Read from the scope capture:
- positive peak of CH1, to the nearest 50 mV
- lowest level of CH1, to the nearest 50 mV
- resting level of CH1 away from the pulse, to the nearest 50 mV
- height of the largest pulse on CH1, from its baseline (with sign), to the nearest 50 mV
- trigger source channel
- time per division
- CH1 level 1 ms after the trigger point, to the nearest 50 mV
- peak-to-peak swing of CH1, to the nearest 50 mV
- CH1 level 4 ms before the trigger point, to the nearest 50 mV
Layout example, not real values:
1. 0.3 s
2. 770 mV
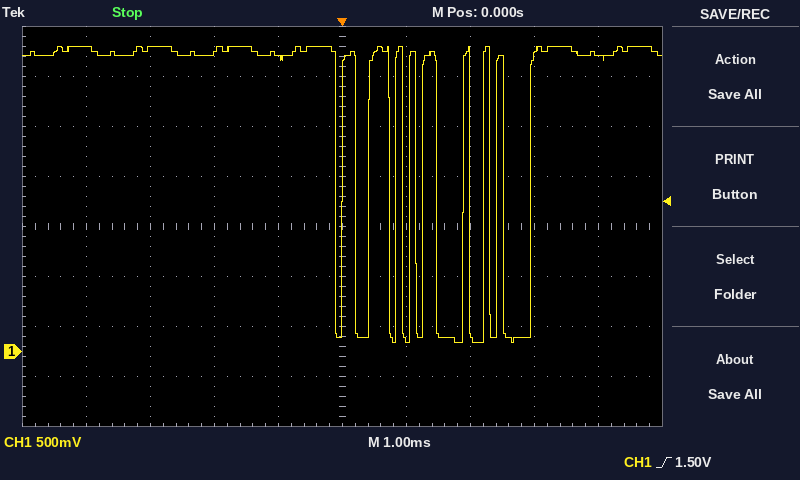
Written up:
1. 3.05 V
2. 100 mV
3. 2.95 V
4. -2.85 V
5. CH1
6. 1 ms
7. 150 mV
8. 2.95 V
9. 3.05 V
